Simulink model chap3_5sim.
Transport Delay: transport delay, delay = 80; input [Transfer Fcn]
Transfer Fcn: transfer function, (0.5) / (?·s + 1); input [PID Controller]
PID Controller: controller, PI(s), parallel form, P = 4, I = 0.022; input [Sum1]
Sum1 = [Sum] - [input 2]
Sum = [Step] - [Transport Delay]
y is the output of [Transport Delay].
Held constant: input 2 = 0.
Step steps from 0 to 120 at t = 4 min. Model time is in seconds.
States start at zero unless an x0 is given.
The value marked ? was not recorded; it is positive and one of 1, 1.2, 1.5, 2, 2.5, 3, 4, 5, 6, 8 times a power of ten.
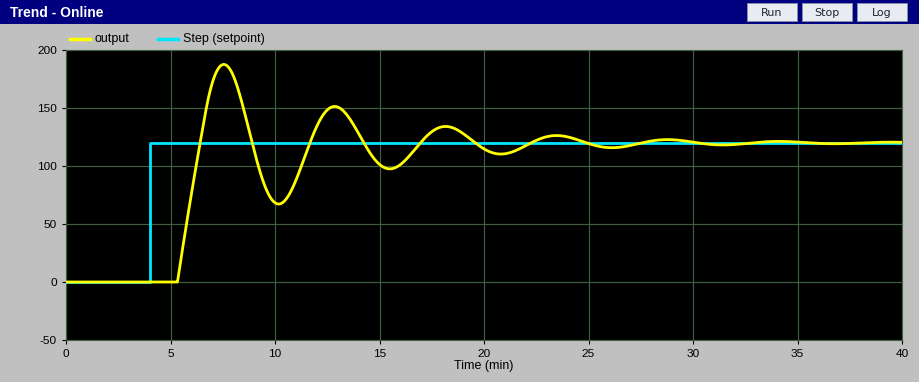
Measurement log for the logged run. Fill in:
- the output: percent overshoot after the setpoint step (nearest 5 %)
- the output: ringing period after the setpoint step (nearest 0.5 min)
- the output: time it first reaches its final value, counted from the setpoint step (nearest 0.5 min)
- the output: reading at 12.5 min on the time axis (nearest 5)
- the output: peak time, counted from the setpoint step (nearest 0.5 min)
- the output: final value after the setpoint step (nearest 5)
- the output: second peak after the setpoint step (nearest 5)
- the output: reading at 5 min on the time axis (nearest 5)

55 %
5.5 min
2.5 min
150
3.5 min
120
150
0
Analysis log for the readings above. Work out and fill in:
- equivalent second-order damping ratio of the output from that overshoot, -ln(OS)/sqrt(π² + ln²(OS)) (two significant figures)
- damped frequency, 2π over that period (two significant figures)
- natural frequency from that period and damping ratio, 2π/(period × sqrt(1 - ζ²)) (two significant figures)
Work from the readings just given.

0.19
1.1 rad/min
1.2 rad/min
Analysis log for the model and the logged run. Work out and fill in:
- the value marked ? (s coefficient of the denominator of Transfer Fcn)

120
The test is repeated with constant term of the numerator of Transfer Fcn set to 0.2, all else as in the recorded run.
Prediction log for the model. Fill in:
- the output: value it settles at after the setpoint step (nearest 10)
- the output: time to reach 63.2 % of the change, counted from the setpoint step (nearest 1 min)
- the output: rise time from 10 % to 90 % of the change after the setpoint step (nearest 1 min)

120
3 min
6 min
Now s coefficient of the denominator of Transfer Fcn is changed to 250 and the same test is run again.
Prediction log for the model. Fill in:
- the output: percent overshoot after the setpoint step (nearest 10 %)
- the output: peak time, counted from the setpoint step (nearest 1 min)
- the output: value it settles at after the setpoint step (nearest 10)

30 %
5 min
120
